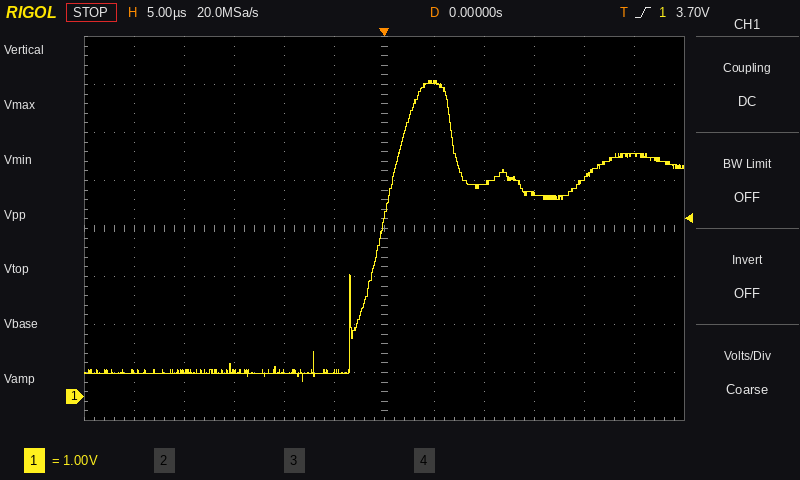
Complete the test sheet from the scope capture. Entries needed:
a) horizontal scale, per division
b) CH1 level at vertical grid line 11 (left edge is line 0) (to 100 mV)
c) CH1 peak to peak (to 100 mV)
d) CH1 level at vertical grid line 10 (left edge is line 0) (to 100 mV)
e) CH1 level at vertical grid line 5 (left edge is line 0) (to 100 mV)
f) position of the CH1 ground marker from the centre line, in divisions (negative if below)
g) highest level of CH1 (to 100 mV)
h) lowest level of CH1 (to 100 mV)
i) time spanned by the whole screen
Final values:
5 µs
5.0 V
6.3 V
4.6 V
500 mV
-3.5 div
6.6 V
300 mV
60 µs
